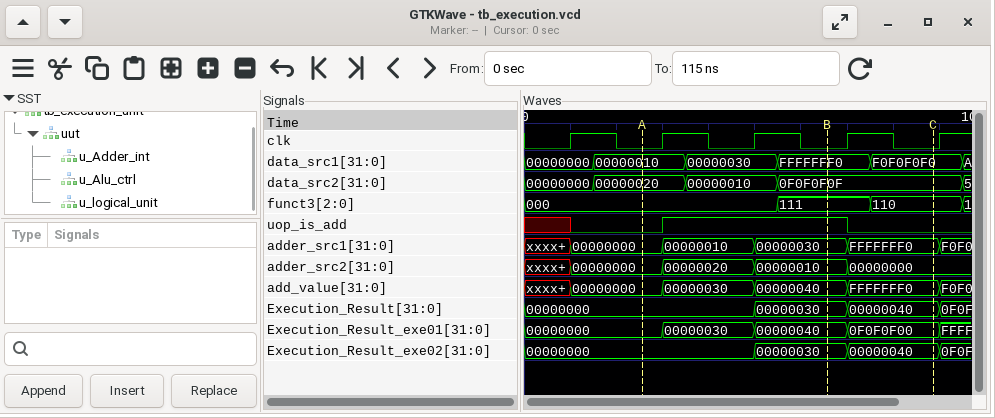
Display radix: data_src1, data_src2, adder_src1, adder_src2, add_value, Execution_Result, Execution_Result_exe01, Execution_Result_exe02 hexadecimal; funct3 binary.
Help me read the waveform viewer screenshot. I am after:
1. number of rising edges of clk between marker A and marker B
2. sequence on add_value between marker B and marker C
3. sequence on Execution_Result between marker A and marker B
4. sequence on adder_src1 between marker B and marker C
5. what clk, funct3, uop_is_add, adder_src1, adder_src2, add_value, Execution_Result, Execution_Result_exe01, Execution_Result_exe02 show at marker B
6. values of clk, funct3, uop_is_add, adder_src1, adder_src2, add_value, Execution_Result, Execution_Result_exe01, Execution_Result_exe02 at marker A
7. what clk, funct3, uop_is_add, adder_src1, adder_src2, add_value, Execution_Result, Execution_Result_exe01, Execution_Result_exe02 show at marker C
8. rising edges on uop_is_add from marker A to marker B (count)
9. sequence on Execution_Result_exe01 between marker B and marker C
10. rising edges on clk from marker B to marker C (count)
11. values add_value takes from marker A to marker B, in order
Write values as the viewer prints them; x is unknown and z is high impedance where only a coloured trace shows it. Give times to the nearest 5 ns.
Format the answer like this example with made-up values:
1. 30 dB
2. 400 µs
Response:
1. 2
2. 00000040, FFFFFFF0
3. 00000000, 00000030
4. 00000030, FFFFFFF0
5. clk=0, funct3=111, uop_is_add=1, adder_src1=00000030, adder_src2=00000010, add_value=00000040, Execution_Result=00000030, Execution_Result_exe01=00000040, Execution_Result_exe02=00000030
6. clk=0, funct3=000, uop_is_add=0, adder_src1=00000000, adder_src2=00000000, add_value=00000000, Execution_Result=00000000, Execution_Result_exe01=00000000, Execution_Result_exe02=00000000
7. clk=0, funct3=110, uop_is_add=0, adder_src1=FFFFFFF0, adder_src2=00000000, add_value=FFFFFFF0, Execution_Result=00000040, Execution_Result_exe01=0F0F0F00, Execution_Result_exe02=00000040
8. 1
9. 00000040, 0F0F0F00
10. 1
11. 00000000, 00000030, 00000040
